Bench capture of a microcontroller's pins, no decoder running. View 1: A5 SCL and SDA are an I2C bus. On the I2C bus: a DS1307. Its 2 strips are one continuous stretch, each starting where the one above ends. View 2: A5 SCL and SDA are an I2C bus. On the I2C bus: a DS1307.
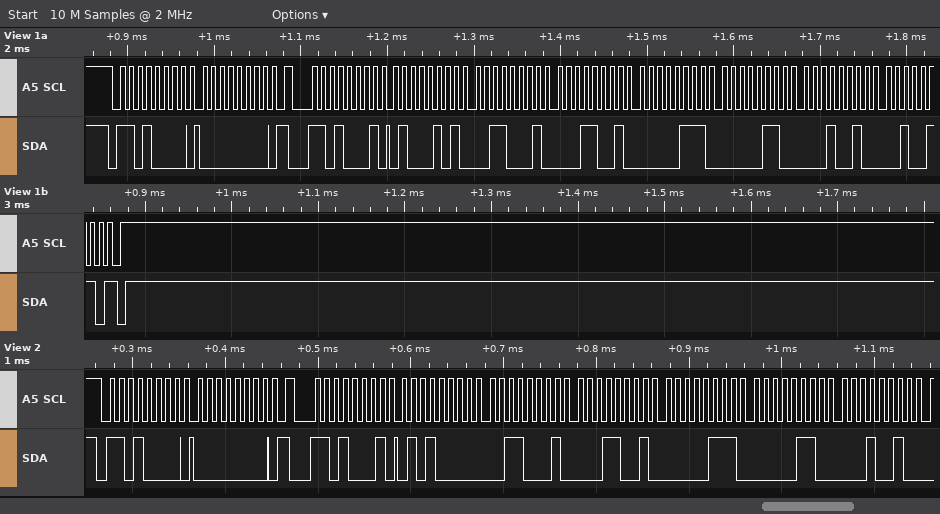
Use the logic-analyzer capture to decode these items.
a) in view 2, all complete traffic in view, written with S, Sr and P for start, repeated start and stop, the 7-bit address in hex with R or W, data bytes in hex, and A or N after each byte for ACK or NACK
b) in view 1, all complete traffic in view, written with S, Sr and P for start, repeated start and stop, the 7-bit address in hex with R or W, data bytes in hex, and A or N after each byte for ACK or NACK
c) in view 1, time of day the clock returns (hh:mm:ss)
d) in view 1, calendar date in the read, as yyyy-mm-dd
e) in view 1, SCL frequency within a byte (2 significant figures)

S 68W A 00 A Sr 68R A 50 A 31 A 19 A 07 A 06 A 12 A
S 68W A 00 A Sr 68R A 45 A 31 A 19 A 07 A 06 A 12 A 26 N P
19:31:45
2026-12-06
100 kHz
